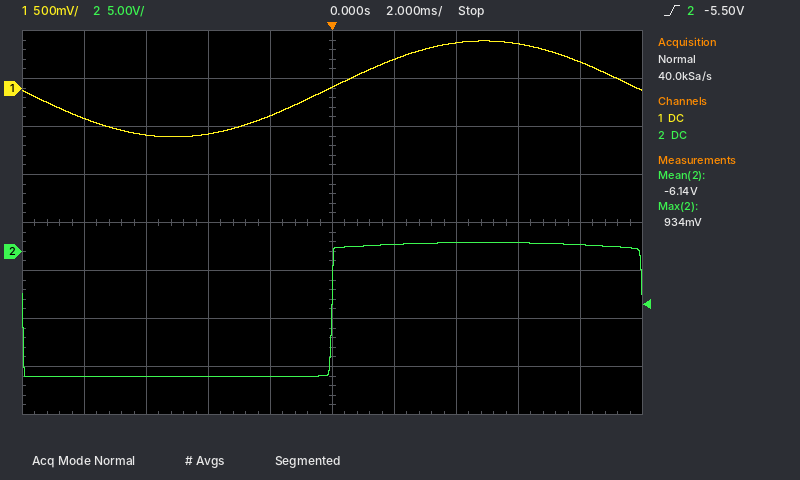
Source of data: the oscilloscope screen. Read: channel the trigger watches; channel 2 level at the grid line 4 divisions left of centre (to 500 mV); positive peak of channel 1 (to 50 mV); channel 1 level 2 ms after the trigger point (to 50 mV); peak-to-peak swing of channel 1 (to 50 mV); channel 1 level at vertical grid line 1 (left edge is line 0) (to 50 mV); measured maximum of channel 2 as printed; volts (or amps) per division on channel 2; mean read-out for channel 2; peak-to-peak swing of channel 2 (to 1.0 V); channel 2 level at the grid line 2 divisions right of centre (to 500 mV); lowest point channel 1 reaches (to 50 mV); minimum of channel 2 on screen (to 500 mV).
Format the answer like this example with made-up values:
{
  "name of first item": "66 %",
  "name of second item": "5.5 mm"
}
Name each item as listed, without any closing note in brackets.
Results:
{
  "channel the trigger watches": "channel 2",
  "channel 2 level at the grid line 4 divisions left of centre": "-13.0 V",
  "positive peak of channel 1": "500 mV",
  "channel 1 level 2 ms after the trigger point": "300 mV",
  "peak-to-peak swing of channel 1": "1.00 V",
  "channel 1 level at vertical grid line 1 (left edge is line 0)": "-300 mV",
  "measured maximum of channel 2 as printed": "934 mV",
  "volts (or amps) per division on channel 2": "5 V",
  "mean read-out for channel 2": "-6.14 V",
  "peak-to-peak swing of channel 2": "14.0 V",
  "channel 2 level at the grid line 2 divisions right of centre": "1.0 V",
  "lowest point channel 1 reaches": "-500 mV",
  "minimum of channel 2 on screen": "-13.0 V"
}
